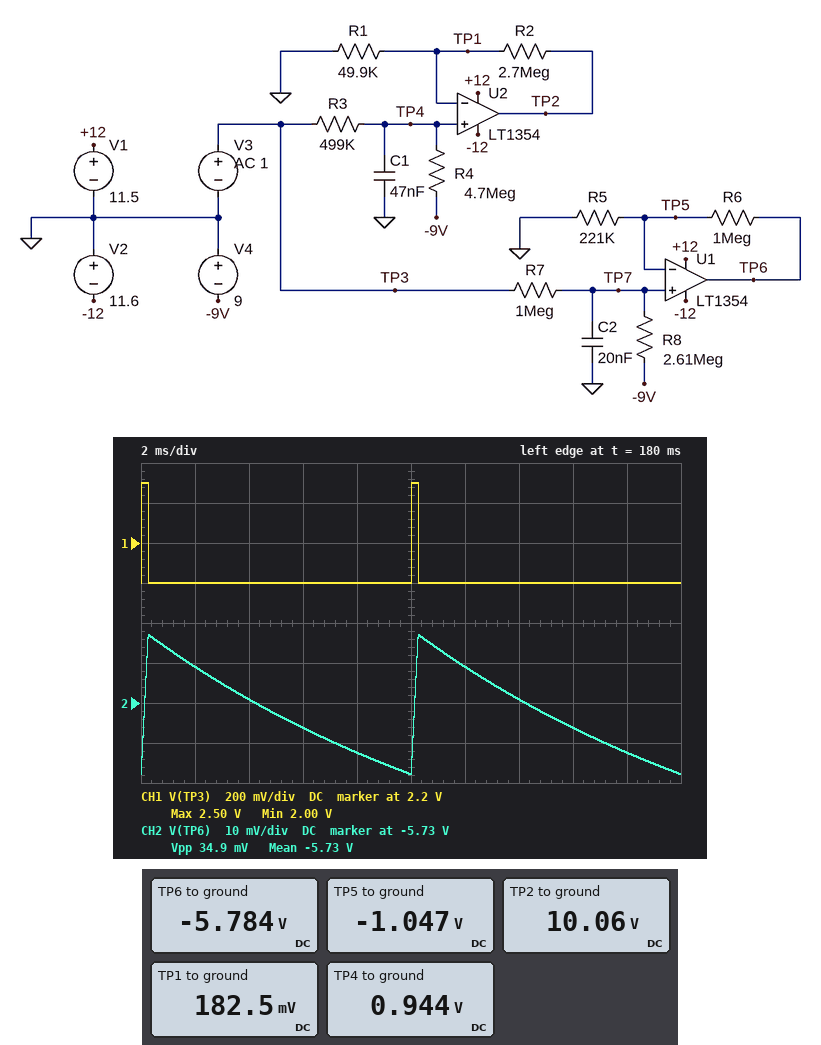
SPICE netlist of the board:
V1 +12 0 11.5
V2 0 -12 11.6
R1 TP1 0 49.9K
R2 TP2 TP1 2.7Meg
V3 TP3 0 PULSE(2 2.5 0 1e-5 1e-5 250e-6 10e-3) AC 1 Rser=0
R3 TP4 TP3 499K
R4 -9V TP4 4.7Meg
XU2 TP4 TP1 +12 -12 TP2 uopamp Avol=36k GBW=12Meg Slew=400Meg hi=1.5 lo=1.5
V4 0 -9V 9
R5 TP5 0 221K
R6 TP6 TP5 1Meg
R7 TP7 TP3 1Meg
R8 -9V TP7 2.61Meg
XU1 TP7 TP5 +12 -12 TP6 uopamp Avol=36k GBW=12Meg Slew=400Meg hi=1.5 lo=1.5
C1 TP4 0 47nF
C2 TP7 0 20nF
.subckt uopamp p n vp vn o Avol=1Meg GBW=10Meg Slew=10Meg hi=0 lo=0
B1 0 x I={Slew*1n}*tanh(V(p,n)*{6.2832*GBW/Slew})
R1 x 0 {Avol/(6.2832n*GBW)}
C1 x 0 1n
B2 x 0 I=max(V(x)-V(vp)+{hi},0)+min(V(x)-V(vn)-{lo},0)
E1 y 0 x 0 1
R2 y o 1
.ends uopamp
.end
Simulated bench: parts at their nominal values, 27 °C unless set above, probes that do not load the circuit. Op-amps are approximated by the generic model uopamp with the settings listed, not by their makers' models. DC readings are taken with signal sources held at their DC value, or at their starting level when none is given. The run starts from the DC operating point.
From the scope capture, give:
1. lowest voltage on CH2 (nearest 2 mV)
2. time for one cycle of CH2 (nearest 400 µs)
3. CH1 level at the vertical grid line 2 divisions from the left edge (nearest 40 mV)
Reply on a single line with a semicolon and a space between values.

-5.748 V; 10.0 ms; 2.00 V
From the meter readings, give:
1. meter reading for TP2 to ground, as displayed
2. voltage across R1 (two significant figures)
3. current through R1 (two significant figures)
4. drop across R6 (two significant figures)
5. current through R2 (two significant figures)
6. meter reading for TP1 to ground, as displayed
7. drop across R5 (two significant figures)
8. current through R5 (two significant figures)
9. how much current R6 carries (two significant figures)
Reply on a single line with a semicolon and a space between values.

10.06 V; 180 mV; 3.7 µA; 4.7 V; 3.7 µA; 182.5 mV; 1.0 V; 4.7 µA; 4.7 µA
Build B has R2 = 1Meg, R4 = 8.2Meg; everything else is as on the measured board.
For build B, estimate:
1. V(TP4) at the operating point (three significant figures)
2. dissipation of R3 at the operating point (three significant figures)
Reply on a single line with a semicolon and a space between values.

1.37 V; 798 nW
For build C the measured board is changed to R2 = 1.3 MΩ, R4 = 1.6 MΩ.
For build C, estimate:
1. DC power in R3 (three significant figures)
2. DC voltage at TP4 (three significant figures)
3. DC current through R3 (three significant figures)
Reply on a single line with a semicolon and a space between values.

13.7 µW; -615 mV; 5.24 µA
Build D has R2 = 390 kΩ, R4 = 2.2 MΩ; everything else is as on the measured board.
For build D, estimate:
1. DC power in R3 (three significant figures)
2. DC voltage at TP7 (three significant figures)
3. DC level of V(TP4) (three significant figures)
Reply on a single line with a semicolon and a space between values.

8.29 µW; -1.05 V; -33.7 mV
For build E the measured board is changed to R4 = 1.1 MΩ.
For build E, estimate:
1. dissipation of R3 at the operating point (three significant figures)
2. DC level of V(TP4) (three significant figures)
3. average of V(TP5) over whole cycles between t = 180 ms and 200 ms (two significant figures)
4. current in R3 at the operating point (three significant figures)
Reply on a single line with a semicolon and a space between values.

23.6 µW; -1.43 V; -1.0 V; 6.88 µA
